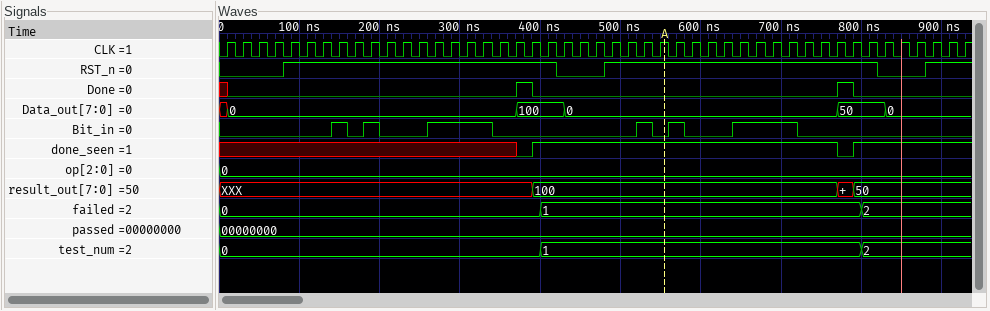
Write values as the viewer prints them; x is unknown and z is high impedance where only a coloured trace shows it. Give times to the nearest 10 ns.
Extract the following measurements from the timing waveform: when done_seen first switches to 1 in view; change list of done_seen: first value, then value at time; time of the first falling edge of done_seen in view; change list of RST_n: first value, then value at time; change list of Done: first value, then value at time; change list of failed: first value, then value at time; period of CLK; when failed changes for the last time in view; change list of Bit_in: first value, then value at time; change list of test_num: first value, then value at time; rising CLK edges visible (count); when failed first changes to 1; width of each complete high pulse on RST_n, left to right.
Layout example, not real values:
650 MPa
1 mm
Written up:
390 ns
x, 0 at 370 ns, 1 at 390 ns, 0 at 770 ns, 1 at 790 ns
770 ns
0, 1 at 80 ns, 0 at 420 ns, 1 at 480 ns, 0 at 820 ns, 1 at 880 ns
x, 0 at 10 ns, 1 at 370 ns, 0 at 390 ns, 1 at 770 ns, 0 at 790 ns
0, 1 at 400 ns, 2 at 800 ns
20 ns
800 ns
0, 1 at 140 ns, 0 at 160 ns, 1 at 180 ns, 0 at 200 ns, 1 at 260 ns, 0 at 340 ns, 1 at 520 ns, 0 at 540 ns, 1 at 560 ns, 0 at 580 ns, 1 at 640 ns, 0 at 720 ns
0, 1 at 400 ns, 2 at 800 ns
47
400 ns
340 ns, 340 ns
